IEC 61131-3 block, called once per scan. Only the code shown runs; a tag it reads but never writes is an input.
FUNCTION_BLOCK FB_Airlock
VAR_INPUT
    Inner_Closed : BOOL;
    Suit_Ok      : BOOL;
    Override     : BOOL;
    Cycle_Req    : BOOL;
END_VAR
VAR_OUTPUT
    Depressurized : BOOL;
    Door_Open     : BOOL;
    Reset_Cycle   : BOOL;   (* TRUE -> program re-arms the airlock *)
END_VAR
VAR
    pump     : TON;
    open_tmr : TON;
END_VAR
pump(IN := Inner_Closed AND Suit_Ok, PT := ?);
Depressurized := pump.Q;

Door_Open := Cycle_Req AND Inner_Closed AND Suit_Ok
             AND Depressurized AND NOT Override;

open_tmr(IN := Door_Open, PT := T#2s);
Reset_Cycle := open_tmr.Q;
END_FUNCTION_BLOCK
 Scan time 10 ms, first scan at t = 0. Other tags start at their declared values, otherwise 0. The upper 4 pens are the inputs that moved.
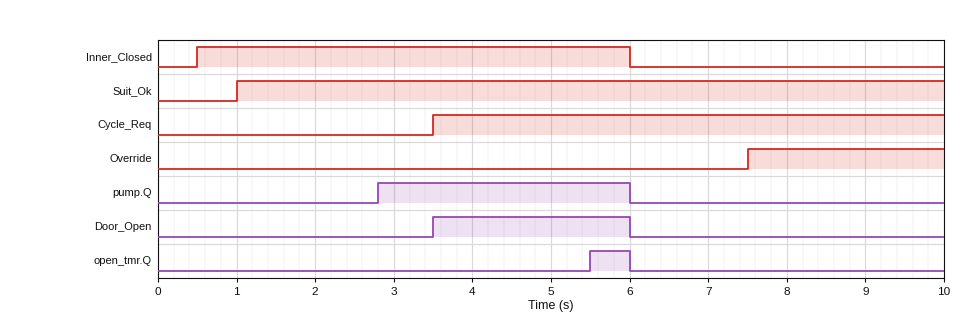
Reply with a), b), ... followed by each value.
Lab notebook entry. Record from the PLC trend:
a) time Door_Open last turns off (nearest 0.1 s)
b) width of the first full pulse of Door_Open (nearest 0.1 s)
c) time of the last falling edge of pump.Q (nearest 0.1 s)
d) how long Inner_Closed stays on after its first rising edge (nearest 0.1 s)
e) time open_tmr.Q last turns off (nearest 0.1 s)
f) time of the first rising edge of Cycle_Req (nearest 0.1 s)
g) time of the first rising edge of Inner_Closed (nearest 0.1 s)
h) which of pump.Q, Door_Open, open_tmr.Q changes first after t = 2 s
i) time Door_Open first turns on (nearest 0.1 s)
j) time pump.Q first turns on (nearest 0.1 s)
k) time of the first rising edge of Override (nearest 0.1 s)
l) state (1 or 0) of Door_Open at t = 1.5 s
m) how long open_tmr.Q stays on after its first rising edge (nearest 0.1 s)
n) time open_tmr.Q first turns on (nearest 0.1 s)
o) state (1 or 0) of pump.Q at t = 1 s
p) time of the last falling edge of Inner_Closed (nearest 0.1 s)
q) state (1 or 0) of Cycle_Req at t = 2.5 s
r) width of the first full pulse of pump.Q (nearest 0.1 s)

a) 6.0 s
b) 2.5 s
c) 6.0 s
d) 5.5 s
e) 6.0 s
f) 3.5 s
g) 0.5 s
h) pump.Q
i) 3.5 s
j) 2.8 s
k) 7.5 s
l) 0
m) 0.5 s
n) 5.5 s
o) 0
p) 6.0 s
q) 0
r) 3.2 s
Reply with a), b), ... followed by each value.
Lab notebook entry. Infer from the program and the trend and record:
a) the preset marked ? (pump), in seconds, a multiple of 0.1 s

a) 1.8 s
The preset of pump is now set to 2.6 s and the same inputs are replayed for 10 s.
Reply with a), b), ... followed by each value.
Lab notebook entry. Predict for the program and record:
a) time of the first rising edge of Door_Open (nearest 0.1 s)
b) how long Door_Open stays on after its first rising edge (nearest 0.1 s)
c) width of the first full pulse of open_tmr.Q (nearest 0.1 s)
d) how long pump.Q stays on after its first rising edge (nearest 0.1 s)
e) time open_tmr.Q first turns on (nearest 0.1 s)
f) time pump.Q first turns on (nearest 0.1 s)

a) 3.6 s
b) 2.4 s
c) 0.4 s
d) 2.4 s
e) 5.6 s
f) 3.6 s
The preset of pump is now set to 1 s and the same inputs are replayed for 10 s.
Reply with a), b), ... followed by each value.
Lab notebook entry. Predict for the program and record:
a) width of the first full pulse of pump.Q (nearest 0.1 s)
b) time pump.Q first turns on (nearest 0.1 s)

a) 4.0 s
b) 2.0 s
